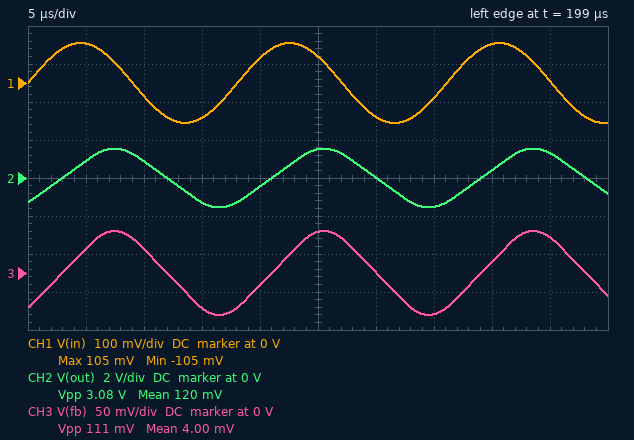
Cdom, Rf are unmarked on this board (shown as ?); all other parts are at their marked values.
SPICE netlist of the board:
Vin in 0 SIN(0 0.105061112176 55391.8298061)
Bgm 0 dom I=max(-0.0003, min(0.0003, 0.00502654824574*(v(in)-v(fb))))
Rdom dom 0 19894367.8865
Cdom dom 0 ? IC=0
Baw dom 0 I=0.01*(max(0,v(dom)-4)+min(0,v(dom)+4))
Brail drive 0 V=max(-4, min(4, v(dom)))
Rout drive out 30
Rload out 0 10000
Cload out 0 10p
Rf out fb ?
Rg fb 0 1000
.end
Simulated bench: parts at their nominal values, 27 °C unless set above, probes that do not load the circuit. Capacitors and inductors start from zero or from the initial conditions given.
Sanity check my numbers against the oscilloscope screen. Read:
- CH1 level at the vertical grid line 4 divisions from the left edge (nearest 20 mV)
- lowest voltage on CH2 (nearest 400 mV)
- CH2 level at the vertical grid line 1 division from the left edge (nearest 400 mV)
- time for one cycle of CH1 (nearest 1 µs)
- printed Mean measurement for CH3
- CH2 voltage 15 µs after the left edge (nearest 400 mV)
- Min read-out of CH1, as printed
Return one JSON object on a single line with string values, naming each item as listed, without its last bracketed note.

{"CH1 level at the vertical grid line 4 divisions from the left edge": "60 mV", "lowest voltage on CH2": "-1.6 V", "CH2 level at the vertical grid line 1 division from the left edge": "800 mV", "time for one cycle of CH1": "18 µs", "printed Mean measurement for CH3": "4.00 mV", "CH2 voltage 15 µs after the left edge": "-1.2 V", "Min read-out of CH1, as printed": "-105 mV"}
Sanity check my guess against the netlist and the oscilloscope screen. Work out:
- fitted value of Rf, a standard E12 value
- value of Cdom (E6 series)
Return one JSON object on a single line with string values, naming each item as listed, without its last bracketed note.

{"fitted value of Rf, a standard E12 value": "27 kΩ", "value of Cdom": "680 pF"}
